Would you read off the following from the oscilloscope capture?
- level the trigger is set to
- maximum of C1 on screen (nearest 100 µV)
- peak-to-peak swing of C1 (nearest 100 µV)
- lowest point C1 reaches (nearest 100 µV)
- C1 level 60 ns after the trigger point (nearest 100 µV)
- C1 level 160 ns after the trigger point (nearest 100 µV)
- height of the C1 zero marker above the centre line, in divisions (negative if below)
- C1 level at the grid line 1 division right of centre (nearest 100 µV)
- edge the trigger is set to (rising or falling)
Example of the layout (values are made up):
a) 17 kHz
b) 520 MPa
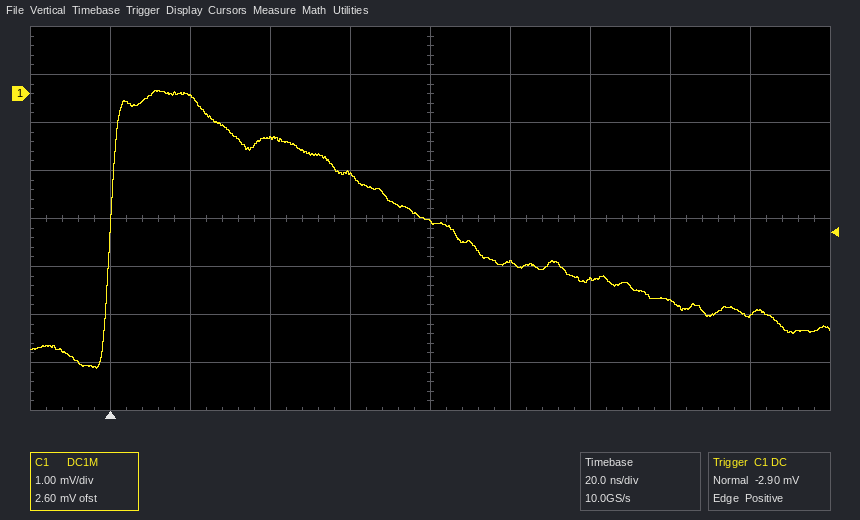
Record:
a) -2.90 mV
b) 100 µV
c) 5.8 mV
d) -5.7 mV
e) -1.7 mV
f) -4.6 mV
g) +2.6 div
h) -3.5 mV
i) rising
